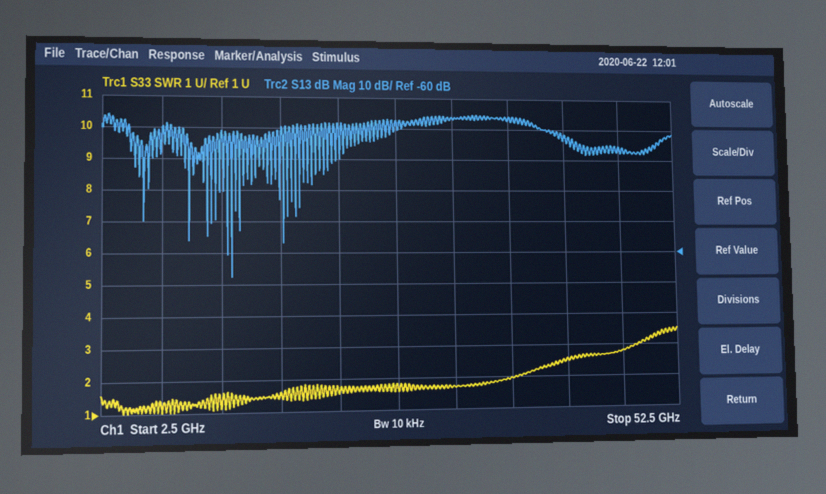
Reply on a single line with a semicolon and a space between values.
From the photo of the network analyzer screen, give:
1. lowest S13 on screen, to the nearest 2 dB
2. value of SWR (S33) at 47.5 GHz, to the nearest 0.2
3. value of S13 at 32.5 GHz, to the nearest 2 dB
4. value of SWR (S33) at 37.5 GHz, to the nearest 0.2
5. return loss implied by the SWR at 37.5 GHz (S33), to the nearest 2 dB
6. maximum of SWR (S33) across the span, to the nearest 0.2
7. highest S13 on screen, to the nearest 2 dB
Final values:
-68 dB; 2.8; -16 dB; 2.0; 10 dB; 3.6; -16 dB
